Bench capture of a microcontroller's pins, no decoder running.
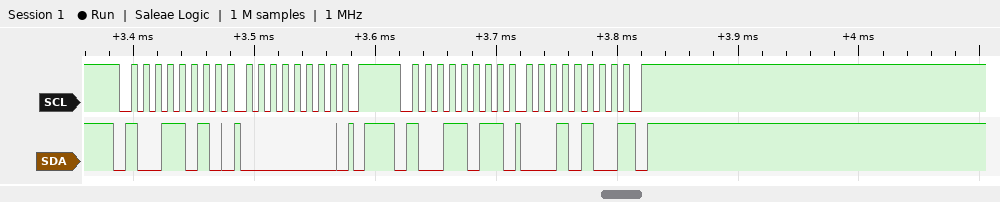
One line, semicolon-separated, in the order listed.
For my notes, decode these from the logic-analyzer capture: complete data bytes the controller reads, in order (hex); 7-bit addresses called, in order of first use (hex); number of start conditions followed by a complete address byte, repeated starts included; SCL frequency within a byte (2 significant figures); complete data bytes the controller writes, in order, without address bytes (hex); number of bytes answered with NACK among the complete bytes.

14; 0x4D; 2; 100 kHz; 00; 1
